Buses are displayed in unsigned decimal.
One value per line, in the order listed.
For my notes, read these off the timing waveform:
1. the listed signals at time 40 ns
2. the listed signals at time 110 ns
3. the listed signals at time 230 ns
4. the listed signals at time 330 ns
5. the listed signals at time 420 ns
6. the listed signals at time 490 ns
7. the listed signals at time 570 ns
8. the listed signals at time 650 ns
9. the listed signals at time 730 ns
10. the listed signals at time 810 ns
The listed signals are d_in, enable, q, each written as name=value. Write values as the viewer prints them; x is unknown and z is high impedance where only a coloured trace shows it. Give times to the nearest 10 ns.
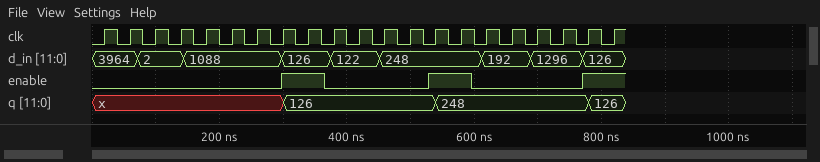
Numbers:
d_in=3964, enable=0, q=x
d_in=2, enable=0, q=x
d_in=1088, enable=0, q=x
d_in=126, enable=1, q=126
d_in=122, enable=0, q=126
d_in=248, enable=0, q=126
d_in=248, enable=1, q=248
d_in=192, enable=0, q=248
d_in=1296, enable=0, q=248
d_in=126, enable=1, q=126
